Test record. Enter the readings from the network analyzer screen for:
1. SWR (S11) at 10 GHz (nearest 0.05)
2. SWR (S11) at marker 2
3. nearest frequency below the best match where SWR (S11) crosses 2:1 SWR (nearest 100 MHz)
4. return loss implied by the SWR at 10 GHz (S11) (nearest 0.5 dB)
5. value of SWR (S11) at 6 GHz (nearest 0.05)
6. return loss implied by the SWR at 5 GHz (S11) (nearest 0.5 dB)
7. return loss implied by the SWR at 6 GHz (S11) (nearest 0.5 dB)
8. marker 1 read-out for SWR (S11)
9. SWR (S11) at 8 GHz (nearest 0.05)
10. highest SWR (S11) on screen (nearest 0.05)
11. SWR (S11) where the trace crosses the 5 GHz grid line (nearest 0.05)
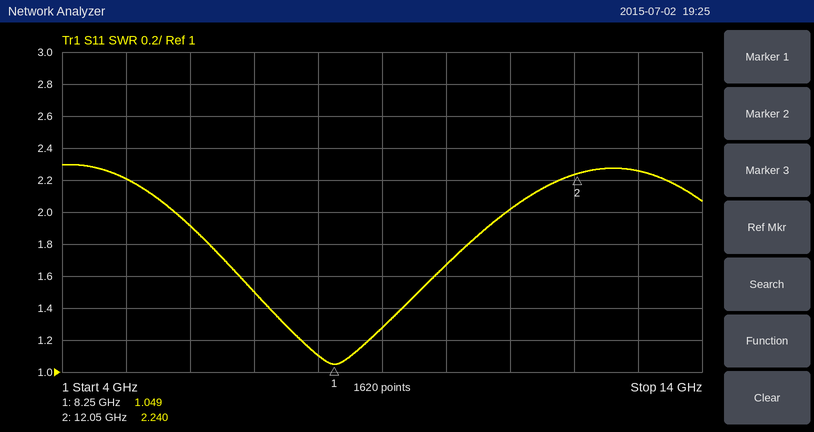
1.65
2.240
5.8 GHz
12.0 dB
1.90
8.5 dB
10.0 dB
1.049
1.10
2.30
2.20
